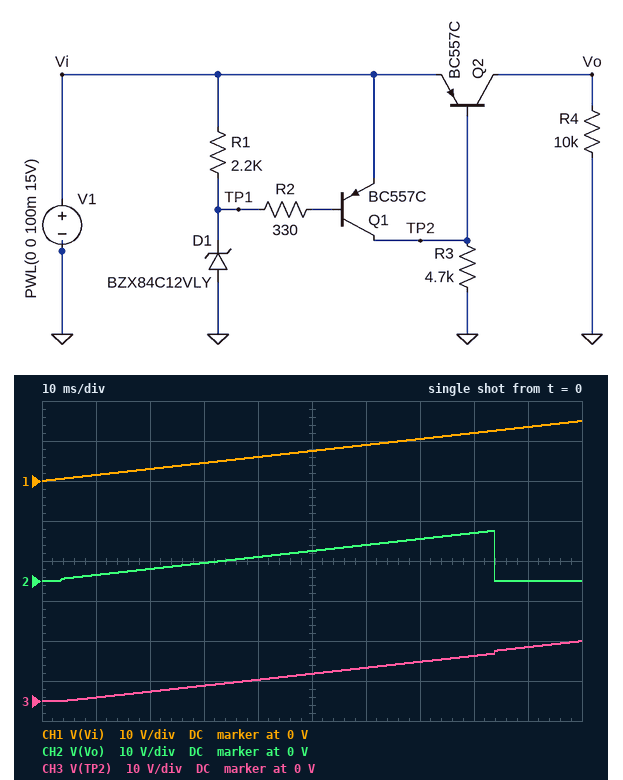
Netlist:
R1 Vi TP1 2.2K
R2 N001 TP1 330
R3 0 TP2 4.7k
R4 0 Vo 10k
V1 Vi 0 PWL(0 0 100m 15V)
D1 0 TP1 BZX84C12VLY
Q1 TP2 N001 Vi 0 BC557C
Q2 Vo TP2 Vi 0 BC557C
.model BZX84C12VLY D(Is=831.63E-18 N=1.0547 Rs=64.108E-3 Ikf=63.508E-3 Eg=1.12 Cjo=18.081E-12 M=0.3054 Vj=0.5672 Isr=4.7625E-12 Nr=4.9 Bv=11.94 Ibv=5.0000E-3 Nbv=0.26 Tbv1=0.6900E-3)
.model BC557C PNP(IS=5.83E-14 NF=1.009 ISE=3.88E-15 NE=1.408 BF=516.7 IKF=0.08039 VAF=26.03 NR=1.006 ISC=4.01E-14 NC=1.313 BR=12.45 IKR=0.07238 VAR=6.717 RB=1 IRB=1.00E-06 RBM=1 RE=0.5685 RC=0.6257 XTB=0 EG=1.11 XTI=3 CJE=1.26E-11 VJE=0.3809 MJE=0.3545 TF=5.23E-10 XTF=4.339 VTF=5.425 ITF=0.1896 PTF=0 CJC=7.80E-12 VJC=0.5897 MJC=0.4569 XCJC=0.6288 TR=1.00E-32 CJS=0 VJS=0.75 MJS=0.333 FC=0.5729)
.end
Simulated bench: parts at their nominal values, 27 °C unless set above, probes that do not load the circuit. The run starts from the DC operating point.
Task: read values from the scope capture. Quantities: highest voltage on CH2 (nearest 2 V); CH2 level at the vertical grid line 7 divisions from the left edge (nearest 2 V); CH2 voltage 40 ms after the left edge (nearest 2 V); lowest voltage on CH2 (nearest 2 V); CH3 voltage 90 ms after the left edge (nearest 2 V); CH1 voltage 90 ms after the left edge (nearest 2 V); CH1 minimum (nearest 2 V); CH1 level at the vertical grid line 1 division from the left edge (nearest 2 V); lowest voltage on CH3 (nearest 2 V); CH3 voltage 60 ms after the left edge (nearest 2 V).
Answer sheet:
12 V
10 V
6 V
0 V
14 V
14 V
0 V
2 V
0 V
8 V
